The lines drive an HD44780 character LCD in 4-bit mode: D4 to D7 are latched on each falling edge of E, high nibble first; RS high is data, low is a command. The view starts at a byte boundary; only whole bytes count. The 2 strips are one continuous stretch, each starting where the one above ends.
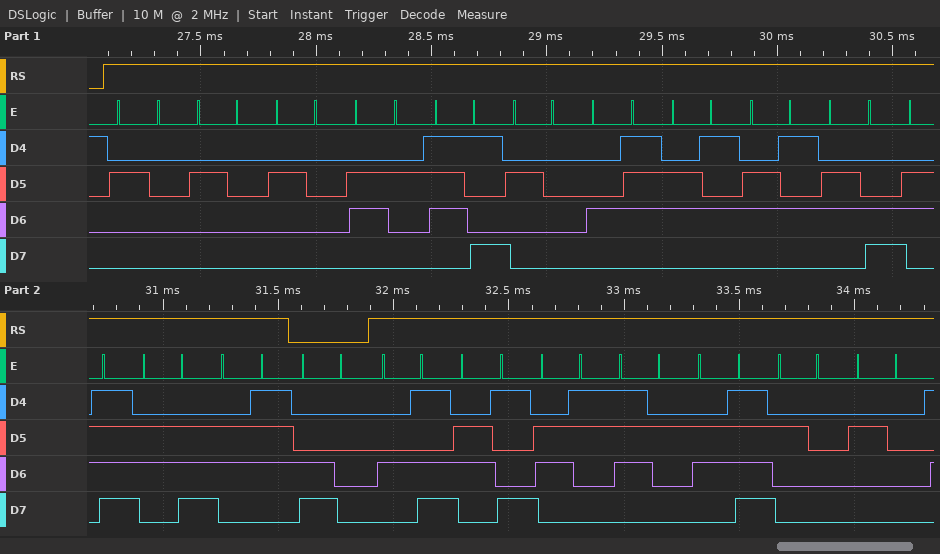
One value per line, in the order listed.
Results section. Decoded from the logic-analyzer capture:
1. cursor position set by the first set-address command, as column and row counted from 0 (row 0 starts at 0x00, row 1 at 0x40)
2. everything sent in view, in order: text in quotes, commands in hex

column 0, row 1
"   by Geelong" 0xC0 "Micro  "
